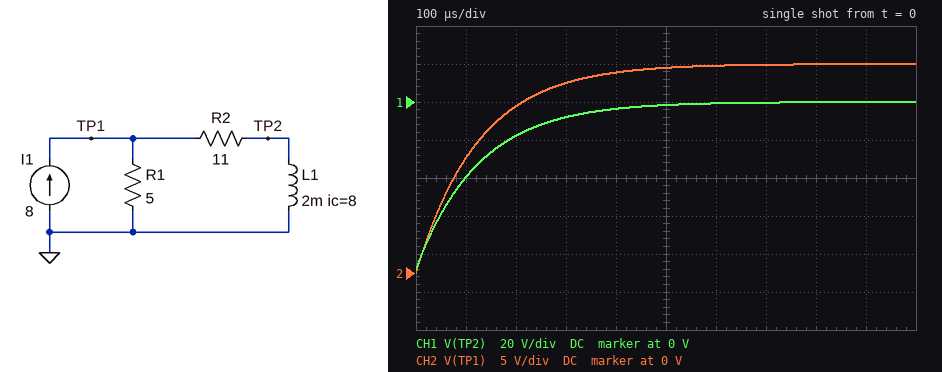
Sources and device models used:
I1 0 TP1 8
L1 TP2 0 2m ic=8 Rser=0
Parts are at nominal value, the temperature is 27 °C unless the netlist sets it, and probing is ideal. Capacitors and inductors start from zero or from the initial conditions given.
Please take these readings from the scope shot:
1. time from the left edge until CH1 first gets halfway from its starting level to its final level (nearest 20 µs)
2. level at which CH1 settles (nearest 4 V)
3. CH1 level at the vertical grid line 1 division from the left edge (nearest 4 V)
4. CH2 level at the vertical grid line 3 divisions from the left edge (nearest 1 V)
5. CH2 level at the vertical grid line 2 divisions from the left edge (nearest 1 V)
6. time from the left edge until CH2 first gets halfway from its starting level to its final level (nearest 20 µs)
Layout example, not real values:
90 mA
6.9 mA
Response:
80 µs
0 V
-40 V
25 V
22 V
80 µs
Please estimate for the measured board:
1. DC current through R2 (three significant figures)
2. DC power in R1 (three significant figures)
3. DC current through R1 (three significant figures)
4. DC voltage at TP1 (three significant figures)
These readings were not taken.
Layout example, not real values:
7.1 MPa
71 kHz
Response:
2.50 A
151 W
5.50 A
27.5 V
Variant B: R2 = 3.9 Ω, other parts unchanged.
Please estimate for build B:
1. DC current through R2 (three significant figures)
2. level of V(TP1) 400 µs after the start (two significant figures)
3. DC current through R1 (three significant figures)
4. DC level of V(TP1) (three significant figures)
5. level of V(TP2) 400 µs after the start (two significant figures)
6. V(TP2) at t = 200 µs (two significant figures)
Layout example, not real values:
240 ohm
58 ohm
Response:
4.49 A
15 V
3.51 A
17.5 V
-5.3 V
-13 V
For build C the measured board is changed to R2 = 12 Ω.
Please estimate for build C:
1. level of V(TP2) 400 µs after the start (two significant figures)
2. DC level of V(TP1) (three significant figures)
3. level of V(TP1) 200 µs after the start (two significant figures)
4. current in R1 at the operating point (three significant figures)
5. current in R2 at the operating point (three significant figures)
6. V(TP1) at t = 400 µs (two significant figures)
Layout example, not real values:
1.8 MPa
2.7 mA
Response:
-3.2 V
28.2 V
23 V
5.65 A
2.35 A
27 V
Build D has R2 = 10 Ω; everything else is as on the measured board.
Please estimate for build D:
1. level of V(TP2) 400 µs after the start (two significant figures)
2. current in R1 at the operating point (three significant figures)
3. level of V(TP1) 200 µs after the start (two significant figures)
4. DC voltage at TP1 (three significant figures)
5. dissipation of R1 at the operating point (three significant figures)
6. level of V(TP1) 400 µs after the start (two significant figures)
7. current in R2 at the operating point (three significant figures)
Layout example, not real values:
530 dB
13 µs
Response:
-4.0 V
5.33 A
21 V
26.7 V
142 W
25 V
2.67 A
